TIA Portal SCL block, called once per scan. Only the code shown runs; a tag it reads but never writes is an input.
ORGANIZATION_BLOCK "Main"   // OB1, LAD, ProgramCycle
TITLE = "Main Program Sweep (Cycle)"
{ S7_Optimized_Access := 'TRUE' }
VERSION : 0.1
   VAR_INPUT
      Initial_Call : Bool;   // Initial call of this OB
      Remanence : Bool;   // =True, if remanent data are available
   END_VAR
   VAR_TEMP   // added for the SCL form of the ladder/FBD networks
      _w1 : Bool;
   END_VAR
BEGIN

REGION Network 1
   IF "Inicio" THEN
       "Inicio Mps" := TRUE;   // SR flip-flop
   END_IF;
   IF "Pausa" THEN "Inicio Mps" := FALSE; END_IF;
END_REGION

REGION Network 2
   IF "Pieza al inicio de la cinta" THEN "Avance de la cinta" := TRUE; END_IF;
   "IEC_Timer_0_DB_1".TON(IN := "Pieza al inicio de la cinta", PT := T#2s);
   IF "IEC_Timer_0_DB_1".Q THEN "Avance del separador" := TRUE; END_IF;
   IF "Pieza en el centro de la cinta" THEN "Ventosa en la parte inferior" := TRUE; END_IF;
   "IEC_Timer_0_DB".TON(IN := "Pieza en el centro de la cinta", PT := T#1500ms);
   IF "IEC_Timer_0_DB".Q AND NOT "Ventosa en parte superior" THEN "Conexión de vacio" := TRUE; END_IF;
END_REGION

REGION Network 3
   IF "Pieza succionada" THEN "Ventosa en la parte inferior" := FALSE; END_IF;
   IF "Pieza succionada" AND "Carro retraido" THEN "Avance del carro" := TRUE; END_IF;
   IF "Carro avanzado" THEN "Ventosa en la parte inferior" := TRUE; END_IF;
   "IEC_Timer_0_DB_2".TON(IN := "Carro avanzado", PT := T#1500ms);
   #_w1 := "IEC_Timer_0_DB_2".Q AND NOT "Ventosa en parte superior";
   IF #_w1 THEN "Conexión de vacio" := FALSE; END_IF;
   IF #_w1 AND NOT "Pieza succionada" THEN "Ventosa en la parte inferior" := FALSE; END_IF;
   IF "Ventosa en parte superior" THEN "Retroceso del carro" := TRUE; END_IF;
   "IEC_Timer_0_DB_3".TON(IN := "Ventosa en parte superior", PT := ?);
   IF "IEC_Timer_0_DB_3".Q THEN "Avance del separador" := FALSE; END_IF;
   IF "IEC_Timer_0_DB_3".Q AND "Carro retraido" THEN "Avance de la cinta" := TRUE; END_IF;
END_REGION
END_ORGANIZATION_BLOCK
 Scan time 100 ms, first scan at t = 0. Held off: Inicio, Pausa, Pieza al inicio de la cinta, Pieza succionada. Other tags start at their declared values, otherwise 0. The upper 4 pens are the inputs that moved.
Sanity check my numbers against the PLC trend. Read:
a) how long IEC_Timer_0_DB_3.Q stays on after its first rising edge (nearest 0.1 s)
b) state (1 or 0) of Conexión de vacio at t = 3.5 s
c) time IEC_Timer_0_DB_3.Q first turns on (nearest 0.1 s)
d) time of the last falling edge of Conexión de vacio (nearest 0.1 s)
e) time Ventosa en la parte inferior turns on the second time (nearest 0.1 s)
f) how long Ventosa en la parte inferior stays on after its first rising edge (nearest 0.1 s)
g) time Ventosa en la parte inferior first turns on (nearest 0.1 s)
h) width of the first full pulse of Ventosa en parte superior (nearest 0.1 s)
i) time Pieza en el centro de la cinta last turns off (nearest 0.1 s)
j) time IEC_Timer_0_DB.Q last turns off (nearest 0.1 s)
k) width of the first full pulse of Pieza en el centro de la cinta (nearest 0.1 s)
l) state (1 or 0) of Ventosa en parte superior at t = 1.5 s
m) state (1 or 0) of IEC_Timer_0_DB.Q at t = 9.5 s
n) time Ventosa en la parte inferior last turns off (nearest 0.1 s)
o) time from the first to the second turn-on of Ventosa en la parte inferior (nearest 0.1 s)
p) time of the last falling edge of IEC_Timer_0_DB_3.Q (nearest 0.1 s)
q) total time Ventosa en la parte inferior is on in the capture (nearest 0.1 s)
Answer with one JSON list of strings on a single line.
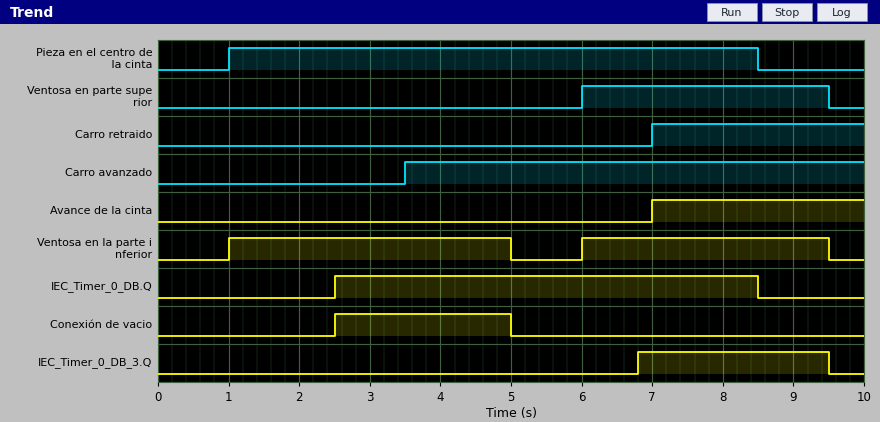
["2.7 s", "1", "6.8 s", "5.0 s", "6.0 s", "4.0 s", "1.0 s", "3.5 s", "8.5 s", "8.5 s", "7.5 s", "0", "0", "9.5 s", "5.0 s", "9.5 s", "7.5 s"]
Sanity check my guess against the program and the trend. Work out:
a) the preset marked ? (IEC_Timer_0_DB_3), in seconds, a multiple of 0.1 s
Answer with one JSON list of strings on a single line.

["0.8 s"]
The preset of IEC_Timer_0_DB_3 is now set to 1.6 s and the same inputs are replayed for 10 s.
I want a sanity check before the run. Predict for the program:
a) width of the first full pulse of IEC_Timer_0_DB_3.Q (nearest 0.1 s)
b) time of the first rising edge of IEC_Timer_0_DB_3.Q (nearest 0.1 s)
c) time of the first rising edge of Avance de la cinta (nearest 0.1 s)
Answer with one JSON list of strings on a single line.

["1.9 s", "7.6 s", "7.6 s"]
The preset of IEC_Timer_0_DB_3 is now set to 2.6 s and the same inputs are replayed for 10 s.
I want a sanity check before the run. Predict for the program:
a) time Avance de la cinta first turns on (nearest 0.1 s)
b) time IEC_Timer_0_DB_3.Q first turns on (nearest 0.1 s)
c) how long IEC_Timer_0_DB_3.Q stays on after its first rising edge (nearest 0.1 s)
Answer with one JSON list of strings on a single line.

["8.6 s", "8.6 s", "0.9 s"]
